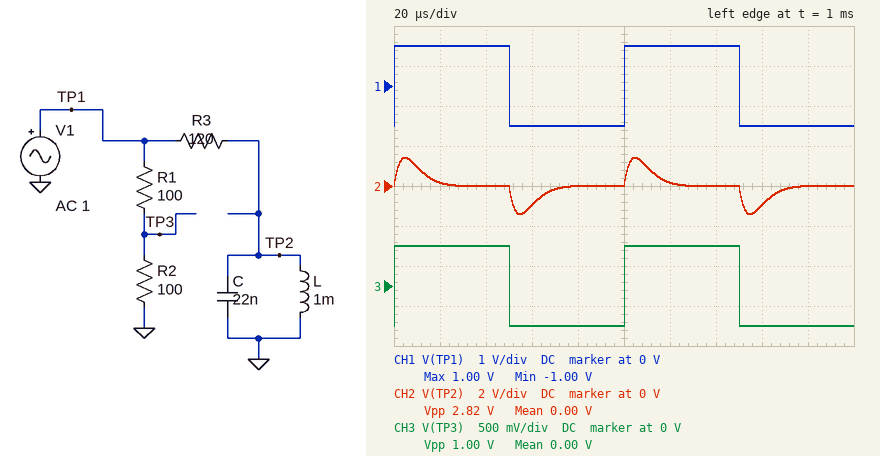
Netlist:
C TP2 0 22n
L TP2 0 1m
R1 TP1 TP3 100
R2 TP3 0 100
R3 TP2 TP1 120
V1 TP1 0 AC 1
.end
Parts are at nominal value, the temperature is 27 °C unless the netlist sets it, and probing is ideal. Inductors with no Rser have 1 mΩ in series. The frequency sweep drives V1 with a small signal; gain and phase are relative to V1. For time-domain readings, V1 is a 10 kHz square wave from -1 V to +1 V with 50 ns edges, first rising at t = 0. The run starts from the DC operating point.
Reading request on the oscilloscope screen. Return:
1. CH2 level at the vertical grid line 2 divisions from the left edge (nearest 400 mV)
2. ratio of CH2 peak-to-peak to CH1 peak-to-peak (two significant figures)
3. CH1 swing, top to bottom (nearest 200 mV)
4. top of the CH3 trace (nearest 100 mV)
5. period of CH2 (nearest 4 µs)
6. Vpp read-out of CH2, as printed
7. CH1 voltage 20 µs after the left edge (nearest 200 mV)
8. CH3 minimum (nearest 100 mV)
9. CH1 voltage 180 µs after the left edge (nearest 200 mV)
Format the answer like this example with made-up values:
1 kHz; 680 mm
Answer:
0 V; 1.4; 2.0 V; 500 mV; 100 µs; 2.82 V; 1.0 V; -500 mV; -1.0 V
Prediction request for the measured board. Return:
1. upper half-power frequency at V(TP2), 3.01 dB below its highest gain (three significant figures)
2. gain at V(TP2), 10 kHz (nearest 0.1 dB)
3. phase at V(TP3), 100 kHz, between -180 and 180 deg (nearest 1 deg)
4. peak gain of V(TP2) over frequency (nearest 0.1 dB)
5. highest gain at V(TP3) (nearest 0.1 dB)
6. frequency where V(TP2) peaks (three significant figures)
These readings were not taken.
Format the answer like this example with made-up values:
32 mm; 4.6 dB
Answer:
75.5 kHz; -6.1 dB; 0 deg; 0 dB; -6.0 dB; 33.9 kHz
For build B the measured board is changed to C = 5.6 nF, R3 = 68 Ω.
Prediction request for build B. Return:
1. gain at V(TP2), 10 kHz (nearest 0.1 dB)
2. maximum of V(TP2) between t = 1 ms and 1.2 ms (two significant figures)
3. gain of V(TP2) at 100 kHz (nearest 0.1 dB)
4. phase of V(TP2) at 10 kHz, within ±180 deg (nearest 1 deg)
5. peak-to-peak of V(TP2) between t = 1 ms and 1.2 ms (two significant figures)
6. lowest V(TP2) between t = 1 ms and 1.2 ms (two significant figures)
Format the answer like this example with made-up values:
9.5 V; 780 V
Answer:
-3.3 dB; 1.8 V; -0.1 dB; 47 deg; 3.6 V; -1.8 V
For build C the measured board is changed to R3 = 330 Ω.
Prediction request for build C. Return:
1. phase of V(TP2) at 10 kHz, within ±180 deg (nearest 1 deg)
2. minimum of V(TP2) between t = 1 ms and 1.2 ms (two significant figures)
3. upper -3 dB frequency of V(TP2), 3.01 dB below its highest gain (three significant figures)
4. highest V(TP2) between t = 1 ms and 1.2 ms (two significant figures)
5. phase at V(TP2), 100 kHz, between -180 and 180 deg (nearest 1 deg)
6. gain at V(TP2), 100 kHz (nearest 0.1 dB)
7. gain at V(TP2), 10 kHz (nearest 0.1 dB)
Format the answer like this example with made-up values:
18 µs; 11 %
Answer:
78 deg; -870 mV; 46.6 kHz; 870 mV; -76 deg; -12.4 dB; -13.8 dB
